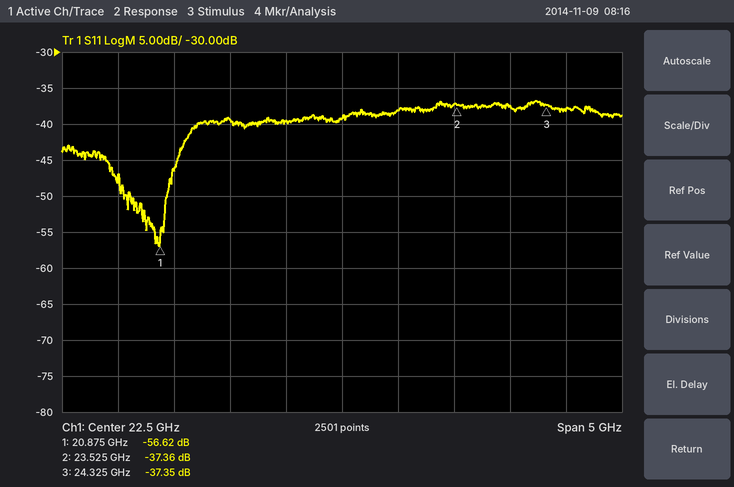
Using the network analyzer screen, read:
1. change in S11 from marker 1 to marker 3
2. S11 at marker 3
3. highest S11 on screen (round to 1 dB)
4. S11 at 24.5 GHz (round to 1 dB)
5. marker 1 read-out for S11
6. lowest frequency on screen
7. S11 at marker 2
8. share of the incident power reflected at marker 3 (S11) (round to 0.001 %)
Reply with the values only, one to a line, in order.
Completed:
19.27 dB
-37.35 dB
-37 dB
-38 dB
-56.62 dB
20 GHz
-37.36 dB
0.018 %
